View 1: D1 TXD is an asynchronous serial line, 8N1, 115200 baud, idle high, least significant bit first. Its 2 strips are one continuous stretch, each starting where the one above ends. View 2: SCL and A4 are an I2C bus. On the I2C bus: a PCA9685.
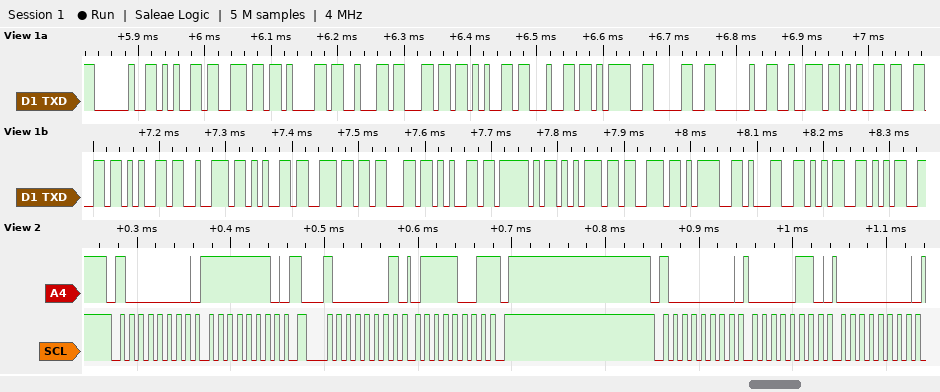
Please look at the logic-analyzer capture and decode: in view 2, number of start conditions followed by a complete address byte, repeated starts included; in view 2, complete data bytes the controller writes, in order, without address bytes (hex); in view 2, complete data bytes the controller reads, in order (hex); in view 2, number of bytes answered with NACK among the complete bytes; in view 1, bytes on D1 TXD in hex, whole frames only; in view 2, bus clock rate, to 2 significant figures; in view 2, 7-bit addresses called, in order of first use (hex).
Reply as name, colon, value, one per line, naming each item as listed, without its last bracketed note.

in view 2, number of start conditions followed by a complete address byte, repeated starts included: 3
in view 2, complete data bytes the controller writes, in order, without address bytes: FE 06 00
in view 2, complete data bytes the controller reads, in order: 79
in view 2, number of bytes answered with NACK among the complete bytes: 1
in view 1, bytes on D1 TXD in hex, whole frames only: 20 65 6E 61 62 6C 65 64 3D 30 20 72 65 66 65 72 65 6E 63 65 5F 75 73 3D 31 35 35
in view 2, bus clock rate, to 2 significant figures: 100 kHz
in view 2, 7-bit addresses called, in order of first use: 0x40
